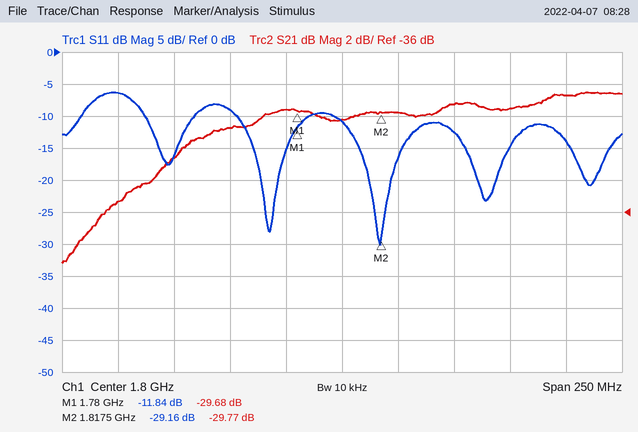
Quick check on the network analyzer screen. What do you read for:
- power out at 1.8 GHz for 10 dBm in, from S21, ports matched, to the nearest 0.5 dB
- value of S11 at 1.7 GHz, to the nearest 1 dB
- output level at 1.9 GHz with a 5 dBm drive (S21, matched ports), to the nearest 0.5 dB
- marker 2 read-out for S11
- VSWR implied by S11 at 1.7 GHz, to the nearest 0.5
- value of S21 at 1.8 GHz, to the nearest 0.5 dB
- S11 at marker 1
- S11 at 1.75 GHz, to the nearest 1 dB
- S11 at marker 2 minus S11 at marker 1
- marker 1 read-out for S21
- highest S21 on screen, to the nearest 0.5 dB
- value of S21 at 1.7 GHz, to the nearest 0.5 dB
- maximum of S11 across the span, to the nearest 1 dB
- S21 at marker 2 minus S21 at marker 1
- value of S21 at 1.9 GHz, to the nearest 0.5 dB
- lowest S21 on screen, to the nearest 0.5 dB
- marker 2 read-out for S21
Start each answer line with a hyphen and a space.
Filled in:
- -20.0 dBm
- -6 dB
- -23.5 dBm
- -29.16 dB
- 3.0
- -30.0 dB
- -11.84 dB
- -9 dB
- -17.32 dB
- -29.68 dB
- -28.5 dB
- -35.5 dB
- -6 dB
- -0.09 dB
- -28.5 dB
- -39.0 dB
- -29.77 dB
